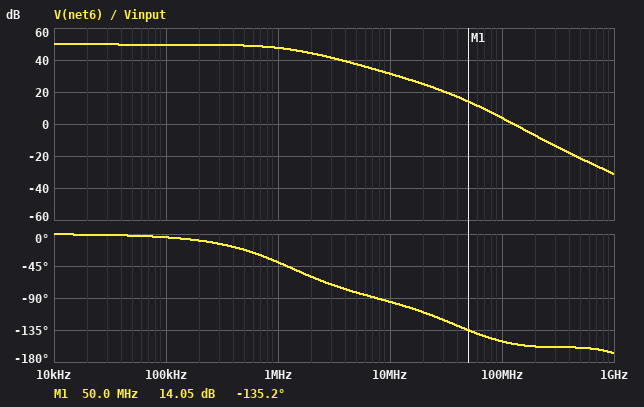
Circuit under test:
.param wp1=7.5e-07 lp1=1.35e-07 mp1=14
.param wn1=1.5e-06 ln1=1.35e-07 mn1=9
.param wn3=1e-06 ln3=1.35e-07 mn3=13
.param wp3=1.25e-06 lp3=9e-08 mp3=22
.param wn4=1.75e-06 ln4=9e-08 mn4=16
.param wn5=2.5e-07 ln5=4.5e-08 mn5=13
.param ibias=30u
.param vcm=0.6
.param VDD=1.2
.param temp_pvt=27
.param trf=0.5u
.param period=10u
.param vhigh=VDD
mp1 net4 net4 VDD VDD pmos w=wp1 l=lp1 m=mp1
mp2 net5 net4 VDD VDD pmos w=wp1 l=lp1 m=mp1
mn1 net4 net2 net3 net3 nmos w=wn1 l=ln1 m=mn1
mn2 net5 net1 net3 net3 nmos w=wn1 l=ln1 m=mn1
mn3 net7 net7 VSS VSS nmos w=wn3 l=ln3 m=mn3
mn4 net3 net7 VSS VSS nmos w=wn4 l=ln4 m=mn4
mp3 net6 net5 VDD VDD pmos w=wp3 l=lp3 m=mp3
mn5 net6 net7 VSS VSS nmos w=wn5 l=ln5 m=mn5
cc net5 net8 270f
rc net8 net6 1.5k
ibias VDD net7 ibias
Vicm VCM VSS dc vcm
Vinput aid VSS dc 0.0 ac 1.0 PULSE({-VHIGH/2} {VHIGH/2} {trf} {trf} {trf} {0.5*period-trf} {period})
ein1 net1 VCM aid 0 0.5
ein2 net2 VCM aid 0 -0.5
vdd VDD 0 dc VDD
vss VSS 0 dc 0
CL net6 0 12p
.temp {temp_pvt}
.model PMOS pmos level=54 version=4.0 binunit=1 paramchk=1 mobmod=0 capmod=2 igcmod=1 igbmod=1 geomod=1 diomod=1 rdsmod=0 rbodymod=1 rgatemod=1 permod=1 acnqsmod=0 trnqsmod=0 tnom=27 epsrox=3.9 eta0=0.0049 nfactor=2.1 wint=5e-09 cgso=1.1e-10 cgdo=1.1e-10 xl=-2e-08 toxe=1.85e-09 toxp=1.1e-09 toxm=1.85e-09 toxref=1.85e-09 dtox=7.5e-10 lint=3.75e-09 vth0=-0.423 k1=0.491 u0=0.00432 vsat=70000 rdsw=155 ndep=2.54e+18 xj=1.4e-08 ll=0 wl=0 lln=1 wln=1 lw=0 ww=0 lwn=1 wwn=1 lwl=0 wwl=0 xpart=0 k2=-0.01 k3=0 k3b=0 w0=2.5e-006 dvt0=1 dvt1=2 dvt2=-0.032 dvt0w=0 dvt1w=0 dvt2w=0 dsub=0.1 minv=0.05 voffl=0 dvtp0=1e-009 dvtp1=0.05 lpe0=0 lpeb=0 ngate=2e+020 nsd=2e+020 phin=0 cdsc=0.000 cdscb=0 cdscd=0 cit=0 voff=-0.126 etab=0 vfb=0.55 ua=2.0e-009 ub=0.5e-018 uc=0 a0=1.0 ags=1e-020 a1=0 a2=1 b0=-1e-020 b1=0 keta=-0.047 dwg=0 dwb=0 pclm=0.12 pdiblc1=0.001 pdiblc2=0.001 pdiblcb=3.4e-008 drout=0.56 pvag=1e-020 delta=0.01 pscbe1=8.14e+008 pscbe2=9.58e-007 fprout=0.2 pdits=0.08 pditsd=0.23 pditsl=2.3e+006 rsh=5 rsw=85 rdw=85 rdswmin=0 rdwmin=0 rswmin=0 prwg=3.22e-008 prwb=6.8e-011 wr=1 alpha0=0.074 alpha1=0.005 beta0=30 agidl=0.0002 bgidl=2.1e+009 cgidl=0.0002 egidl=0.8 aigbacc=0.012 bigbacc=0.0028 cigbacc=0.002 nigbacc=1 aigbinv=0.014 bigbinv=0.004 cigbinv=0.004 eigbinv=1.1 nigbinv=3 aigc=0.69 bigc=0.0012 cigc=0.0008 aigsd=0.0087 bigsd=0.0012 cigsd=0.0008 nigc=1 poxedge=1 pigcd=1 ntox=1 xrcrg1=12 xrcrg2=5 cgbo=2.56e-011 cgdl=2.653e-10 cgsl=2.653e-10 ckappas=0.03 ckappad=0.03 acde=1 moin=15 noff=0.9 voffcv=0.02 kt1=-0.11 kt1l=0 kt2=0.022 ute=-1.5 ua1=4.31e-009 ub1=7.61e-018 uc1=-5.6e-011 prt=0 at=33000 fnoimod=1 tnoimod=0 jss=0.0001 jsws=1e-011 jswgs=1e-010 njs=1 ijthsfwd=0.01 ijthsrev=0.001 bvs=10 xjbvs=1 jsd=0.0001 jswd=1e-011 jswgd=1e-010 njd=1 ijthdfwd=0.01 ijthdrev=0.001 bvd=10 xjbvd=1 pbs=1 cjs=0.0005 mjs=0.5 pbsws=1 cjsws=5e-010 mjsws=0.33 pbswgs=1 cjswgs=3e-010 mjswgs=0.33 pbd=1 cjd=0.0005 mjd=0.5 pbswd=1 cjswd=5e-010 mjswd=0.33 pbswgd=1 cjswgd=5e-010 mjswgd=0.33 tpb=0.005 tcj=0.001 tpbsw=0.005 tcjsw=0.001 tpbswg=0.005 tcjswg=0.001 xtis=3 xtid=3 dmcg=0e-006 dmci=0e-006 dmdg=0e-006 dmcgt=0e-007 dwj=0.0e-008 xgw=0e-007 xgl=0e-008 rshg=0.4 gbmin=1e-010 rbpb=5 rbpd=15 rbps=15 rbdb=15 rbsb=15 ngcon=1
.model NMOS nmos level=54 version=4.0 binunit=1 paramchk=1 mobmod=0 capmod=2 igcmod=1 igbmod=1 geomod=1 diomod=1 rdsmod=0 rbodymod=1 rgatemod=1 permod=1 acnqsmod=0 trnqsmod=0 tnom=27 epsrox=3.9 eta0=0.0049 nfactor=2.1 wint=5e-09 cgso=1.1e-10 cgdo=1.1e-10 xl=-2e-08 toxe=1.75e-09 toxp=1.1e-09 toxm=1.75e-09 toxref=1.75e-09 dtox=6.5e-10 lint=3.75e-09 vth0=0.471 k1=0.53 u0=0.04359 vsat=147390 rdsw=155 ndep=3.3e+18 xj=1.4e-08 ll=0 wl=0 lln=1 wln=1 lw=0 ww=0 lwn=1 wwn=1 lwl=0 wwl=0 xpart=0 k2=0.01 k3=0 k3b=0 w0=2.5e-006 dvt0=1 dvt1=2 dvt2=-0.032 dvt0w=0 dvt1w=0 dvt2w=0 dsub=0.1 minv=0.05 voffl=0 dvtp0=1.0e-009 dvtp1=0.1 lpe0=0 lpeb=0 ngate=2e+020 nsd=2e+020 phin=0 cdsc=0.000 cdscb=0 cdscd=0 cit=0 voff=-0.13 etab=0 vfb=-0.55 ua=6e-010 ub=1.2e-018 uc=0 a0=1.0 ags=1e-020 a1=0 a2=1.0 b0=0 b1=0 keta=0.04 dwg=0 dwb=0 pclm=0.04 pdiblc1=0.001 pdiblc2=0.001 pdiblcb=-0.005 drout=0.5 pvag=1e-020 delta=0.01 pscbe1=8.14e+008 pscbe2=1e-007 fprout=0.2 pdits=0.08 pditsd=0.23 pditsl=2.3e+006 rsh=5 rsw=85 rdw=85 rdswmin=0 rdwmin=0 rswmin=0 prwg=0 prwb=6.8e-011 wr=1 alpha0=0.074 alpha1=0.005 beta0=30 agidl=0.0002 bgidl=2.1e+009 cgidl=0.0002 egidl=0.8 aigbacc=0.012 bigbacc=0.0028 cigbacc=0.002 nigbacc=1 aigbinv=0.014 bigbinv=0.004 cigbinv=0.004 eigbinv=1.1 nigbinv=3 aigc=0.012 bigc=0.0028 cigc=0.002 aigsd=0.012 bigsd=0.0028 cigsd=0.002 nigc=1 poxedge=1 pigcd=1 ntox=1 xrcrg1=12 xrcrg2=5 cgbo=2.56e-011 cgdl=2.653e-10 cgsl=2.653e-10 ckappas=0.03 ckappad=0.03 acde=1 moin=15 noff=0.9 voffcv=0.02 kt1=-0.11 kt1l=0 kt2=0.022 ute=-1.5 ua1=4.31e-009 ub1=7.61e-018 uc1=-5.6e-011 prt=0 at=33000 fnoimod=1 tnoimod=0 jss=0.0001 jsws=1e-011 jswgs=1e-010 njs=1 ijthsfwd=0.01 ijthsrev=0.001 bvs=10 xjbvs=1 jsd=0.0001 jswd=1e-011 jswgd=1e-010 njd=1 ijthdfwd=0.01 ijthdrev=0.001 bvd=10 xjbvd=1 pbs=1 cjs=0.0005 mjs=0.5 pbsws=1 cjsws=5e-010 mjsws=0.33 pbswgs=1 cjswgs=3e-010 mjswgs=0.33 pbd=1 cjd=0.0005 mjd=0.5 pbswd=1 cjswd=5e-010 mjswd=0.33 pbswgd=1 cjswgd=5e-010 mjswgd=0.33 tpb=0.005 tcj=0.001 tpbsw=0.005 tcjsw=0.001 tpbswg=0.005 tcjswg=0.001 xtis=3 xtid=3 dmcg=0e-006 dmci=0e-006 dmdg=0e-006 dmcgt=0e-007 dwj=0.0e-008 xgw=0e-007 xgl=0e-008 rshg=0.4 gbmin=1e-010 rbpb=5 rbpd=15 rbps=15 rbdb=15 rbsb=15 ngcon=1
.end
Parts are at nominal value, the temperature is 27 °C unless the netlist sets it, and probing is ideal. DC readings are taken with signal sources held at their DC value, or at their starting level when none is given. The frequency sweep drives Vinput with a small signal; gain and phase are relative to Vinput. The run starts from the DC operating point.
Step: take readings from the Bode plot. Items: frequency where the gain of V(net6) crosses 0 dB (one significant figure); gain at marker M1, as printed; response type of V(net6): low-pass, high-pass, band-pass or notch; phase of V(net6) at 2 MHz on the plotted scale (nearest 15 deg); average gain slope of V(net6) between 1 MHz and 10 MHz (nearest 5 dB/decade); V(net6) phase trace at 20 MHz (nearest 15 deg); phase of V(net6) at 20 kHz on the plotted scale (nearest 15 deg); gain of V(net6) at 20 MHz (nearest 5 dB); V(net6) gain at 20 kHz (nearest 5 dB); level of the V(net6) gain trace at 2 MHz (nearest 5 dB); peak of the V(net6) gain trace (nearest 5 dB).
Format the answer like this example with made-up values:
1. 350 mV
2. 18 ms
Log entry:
1. 100 MHz
2. 14.05 dB
3. low-pass
4. -60 deg
5. -15 dB/decade
6. -105 deg
7. 0 deg
8. 25 dB
9. 50 dB
10. 45 dB
11. 50 dB
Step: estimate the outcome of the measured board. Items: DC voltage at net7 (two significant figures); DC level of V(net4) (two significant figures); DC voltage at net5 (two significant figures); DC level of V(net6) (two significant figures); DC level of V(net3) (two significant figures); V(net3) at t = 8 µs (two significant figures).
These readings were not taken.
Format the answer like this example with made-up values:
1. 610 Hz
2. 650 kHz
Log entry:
1. 400 mV
2. 630 mV
3. 630 mV
4. 690 mV
5. 170 mV
6. 420 mV
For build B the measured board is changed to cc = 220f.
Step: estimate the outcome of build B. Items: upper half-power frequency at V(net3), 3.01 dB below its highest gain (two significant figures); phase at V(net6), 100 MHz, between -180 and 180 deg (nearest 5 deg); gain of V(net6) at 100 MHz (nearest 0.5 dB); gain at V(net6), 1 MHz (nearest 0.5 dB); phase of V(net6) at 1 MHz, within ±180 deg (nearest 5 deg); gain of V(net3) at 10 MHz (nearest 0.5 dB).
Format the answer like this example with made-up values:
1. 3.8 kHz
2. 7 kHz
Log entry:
1. 1.5 MHz
2. -155 deg
3. 5.0 dB
4. 48.0 dB
5. -35 deg
6. -24.5 dB
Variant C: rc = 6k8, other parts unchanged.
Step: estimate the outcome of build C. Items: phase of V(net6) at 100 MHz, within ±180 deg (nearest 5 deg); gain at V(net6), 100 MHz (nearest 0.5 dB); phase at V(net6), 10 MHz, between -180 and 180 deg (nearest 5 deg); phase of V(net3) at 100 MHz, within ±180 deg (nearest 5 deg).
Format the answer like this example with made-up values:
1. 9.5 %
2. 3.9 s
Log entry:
1. -125 deg
2. 7.0 dB
3. -90 deg
4. 160 deg
